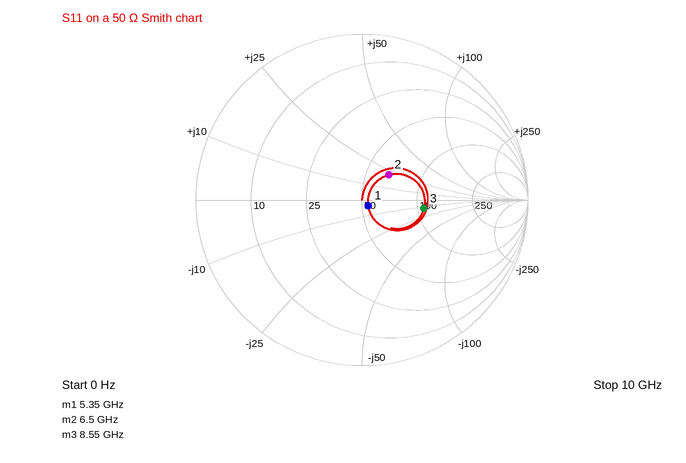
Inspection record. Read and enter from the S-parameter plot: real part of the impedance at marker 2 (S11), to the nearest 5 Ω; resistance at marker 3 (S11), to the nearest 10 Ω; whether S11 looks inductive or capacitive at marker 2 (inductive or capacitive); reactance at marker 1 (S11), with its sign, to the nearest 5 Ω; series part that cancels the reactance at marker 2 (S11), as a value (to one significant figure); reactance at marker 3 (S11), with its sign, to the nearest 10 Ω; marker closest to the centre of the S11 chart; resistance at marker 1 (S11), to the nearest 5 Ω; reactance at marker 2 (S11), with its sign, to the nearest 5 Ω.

65 Ω
110 Ω
inductive
-5 Ω
1 pF
-10 Ω
marker 1
55 Ω
+20 Ω
